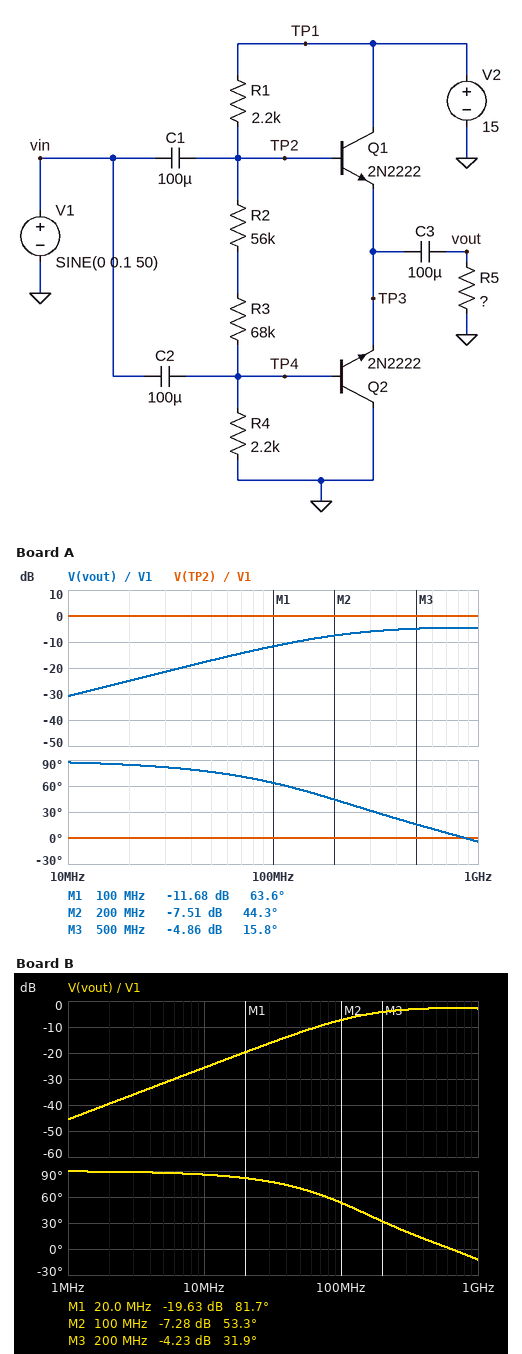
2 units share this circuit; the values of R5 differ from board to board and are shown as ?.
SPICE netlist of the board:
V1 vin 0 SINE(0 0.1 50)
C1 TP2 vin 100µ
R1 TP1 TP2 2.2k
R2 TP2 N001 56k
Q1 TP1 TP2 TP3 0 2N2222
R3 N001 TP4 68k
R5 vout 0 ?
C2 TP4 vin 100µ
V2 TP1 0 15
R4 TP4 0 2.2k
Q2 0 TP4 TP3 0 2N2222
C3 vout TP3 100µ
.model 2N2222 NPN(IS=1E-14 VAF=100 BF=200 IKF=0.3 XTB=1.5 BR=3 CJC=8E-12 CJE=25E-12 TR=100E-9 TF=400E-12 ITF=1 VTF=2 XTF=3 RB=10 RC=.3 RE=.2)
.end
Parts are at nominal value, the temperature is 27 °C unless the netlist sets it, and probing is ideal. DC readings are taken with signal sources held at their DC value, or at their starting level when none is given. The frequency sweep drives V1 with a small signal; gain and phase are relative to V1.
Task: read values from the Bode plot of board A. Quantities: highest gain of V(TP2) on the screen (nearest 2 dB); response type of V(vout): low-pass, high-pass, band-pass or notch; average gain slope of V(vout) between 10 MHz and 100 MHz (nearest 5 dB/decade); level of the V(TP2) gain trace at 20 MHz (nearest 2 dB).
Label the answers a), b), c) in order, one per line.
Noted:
a) 0 dB
b) high-pass
c) 20 dB/decade
d) 0 dB
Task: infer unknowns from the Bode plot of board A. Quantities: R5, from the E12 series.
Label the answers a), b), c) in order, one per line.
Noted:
a) 12 Ω
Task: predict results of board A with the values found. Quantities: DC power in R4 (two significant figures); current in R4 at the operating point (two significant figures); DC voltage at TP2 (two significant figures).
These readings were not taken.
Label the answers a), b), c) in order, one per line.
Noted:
a) 30 µW
b) 120 µA
c) 15 V
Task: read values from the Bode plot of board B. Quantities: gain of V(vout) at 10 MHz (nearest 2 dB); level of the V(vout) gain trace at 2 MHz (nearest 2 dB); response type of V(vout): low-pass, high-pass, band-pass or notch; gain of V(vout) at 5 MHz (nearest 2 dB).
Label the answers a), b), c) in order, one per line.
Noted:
a) -26 dB
b) -40 dB
c) high-pass
d) -32 dB
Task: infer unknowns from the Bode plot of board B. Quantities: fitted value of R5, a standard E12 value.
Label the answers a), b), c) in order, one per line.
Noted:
a) 22 Ω
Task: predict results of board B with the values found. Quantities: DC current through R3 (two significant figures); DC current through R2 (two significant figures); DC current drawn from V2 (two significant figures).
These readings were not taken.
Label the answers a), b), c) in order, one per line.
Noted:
a) 120 µA
b) 120 µA
c) 120 µA
